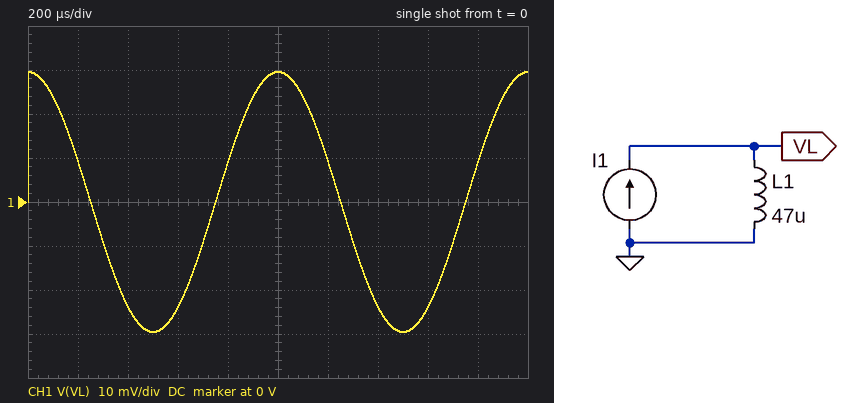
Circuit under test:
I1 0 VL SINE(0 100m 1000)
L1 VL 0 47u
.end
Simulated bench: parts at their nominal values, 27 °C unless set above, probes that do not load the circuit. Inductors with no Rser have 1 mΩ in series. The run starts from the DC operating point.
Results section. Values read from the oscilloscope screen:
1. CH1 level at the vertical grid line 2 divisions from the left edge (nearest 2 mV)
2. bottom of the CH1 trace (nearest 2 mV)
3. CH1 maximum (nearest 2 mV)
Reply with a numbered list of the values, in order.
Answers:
1. -24 mV
2. -30 mV
3. 30 mV
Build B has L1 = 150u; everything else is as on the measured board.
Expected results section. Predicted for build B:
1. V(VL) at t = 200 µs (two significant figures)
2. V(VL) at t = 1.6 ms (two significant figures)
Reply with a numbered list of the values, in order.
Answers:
1. 29 mV
2. -76 mV
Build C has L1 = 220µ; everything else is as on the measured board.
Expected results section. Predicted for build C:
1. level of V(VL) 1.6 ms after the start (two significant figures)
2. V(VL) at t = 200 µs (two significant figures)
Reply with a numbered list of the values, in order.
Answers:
1. -110 mV
2. 43 mV
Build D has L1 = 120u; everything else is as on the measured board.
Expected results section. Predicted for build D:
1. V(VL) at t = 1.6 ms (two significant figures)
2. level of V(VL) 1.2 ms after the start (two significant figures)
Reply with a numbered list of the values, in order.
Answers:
1. -61 mV
2. 23 mV
